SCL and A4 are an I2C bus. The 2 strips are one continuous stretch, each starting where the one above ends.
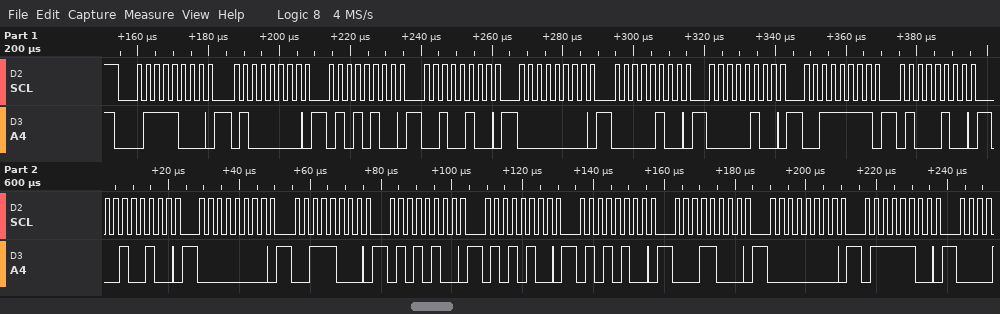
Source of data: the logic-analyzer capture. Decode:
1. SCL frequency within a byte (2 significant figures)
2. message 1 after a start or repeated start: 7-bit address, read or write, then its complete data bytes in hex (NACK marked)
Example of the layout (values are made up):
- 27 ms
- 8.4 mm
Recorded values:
- 400 kHz
- 0x3C write: 40 54 24 00 04 04 3F 44 24 00 38 54 54 54 18 00 7C
